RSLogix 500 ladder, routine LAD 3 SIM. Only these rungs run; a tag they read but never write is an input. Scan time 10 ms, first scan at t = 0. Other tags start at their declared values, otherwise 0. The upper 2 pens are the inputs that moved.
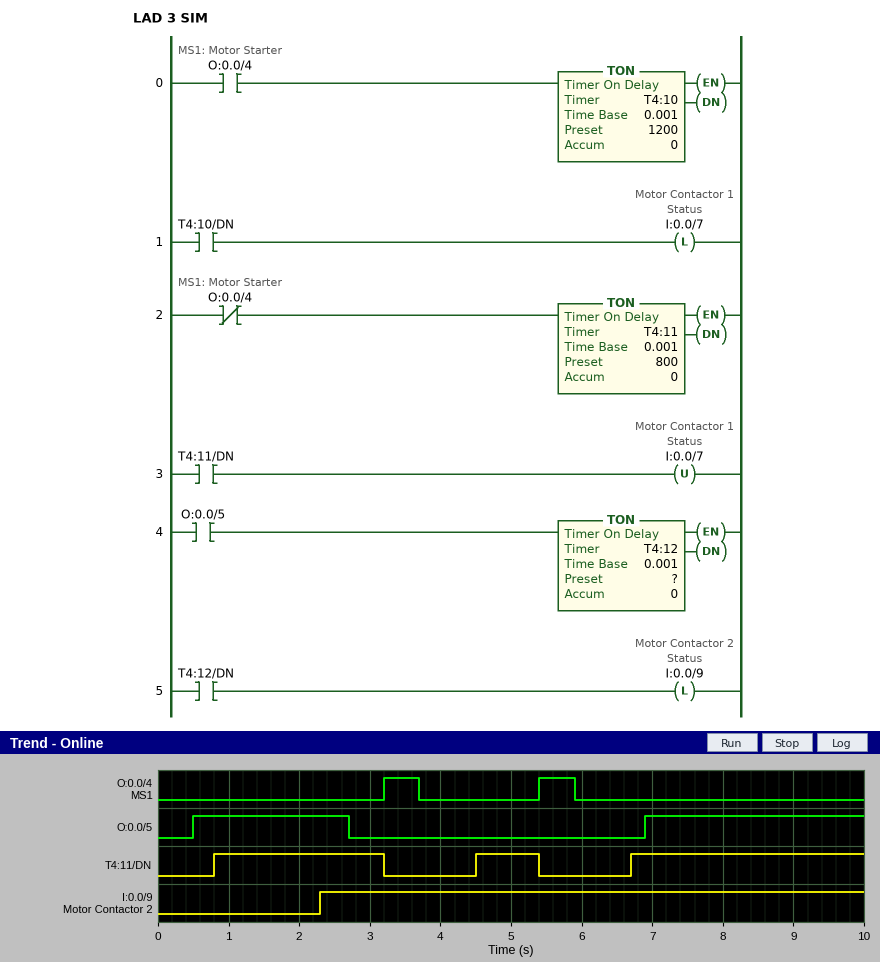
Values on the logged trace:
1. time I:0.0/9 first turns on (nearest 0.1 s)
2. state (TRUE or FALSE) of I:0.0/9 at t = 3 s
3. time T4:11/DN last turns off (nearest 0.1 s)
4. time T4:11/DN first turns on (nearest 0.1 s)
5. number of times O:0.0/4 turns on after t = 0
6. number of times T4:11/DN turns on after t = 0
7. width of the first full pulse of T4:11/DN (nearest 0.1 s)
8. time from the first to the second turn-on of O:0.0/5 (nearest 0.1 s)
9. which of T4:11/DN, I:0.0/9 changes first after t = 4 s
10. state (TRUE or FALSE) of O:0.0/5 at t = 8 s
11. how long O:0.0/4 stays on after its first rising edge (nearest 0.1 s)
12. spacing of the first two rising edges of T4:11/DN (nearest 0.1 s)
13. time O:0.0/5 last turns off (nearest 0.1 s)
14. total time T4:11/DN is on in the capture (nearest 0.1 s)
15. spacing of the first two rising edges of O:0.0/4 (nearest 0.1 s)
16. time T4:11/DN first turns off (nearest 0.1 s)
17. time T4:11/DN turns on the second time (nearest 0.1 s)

2.3 s
TRUE
5.4 s
0.8 s
2
3
2.4 s
6.4 s
T4:11/DN
TRUE
0.5 s
3.7 s
2.7 s
6.6 s
2.2 s
3.2 s
4.5 s
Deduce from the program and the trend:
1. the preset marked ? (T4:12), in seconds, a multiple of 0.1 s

1.8 s
